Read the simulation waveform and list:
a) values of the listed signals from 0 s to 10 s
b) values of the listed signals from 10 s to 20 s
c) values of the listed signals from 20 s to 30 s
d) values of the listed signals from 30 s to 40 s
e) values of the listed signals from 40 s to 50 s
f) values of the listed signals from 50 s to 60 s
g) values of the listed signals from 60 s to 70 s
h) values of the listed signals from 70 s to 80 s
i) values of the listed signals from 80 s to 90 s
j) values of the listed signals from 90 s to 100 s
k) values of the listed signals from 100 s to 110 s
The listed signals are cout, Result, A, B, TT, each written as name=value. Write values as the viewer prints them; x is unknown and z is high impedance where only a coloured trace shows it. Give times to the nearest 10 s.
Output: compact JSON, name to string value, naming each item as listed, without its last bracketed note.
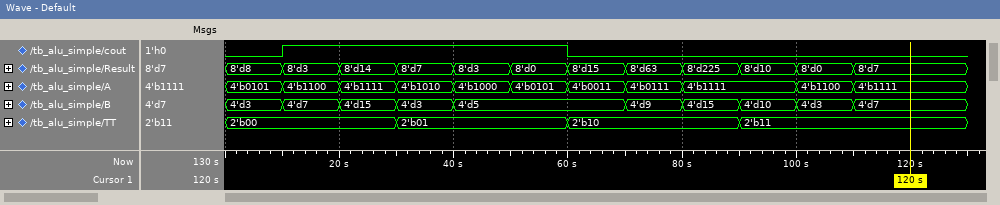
{"values of the listed signals from 0 s to 10 s": "cout=0, Result=8'd8, A=4'b0101, B=4'd3, TT=2'b00", "values of the listed signals from 10 s to 20 s": "cout=1, Result=8'd3, A=4'b1100, B=4'd7, TT=2'b00", "values of the listed signals from 20 s to 30 s": "cout=1, Result=8'd14, A=4'b1111, B=4'd15, TT=2'b00", "values of the listed signals from 30 s to 40 s": "cout=1, Result=8'd7, A=4'b1010, B=4'd3, TT=2'b01", "values of the listed signals from 40 s to 50 s": "cout=1, Result=8'd3, A=4'b1000, B=4'd5, TT=2'b01", "values of the listed signals from 50 s to 60 s": "cout=1, Result=8'd0, A=4'b0101, B=4'd5, TT=2'b01", "values of the listed signals from 60 s to 70 s": "cout=0, Result=8'd15, A=4'b0011, B=4'd5, TT=2'b10", "values of the listed signals from 70 s to 80 s": "cout=0, Result=8'd63, A=4'b0111, B=4'd9, TT=2'b10", "values of the listed signals from 80 s to 90 s": "cout=0, Result=8'd225, A=4'b1111, B=4'd15, TT=2'b10", "values of the listed signals from 90 s to 100 s": "cout=0, Result=8'd10, A=4'b1111, B=4'd10, TT=2'b11", "values of the listed signals from 100 s to 110 s": "cout=0, Result=8'd0, A=4'b1100, B=4'd3, TT=2'b11"}
